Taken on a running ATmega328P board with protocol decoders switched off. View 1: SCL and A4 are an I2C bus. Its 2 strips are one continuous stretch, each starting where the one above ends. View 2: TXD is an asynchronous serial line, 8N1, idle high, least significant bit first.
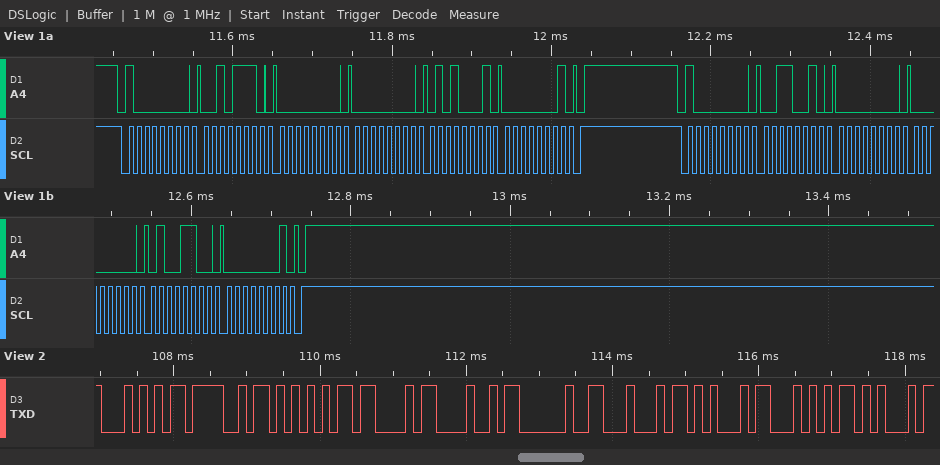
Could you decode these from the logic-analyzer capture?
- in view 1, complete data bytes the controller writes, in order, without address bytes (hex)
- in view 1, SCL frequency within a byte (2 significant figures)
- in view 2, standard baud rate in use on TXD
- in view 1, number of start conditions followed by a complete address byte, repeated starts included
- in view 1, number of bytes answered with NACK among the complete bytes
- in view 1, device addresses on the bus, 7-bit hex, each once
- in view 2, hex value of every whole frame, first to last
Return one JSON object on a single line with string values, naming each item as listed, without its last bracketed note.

{"in view 1, complete data bytes the controller writes, in order, without address bytes": "2E 00 00 51 01 32 00 00 4C 01", "in view 1, SCL frequency within a byte": "100 kHz", "in view 2, standard baud rate in use on TXD": "9600 baud", "in view 1, number of start conditions followed by a complete address byte, repeated starts included": "2", "in view 1, number of bytes answered with NACK among the complete bytes": "0", "in view 1, device addresses on the bus, 7-bit hex, each once": "0x40", "in view 2, hex value of every whole frame, first to last": "54 4F 55 43 48 20 44 45 54 45"}
